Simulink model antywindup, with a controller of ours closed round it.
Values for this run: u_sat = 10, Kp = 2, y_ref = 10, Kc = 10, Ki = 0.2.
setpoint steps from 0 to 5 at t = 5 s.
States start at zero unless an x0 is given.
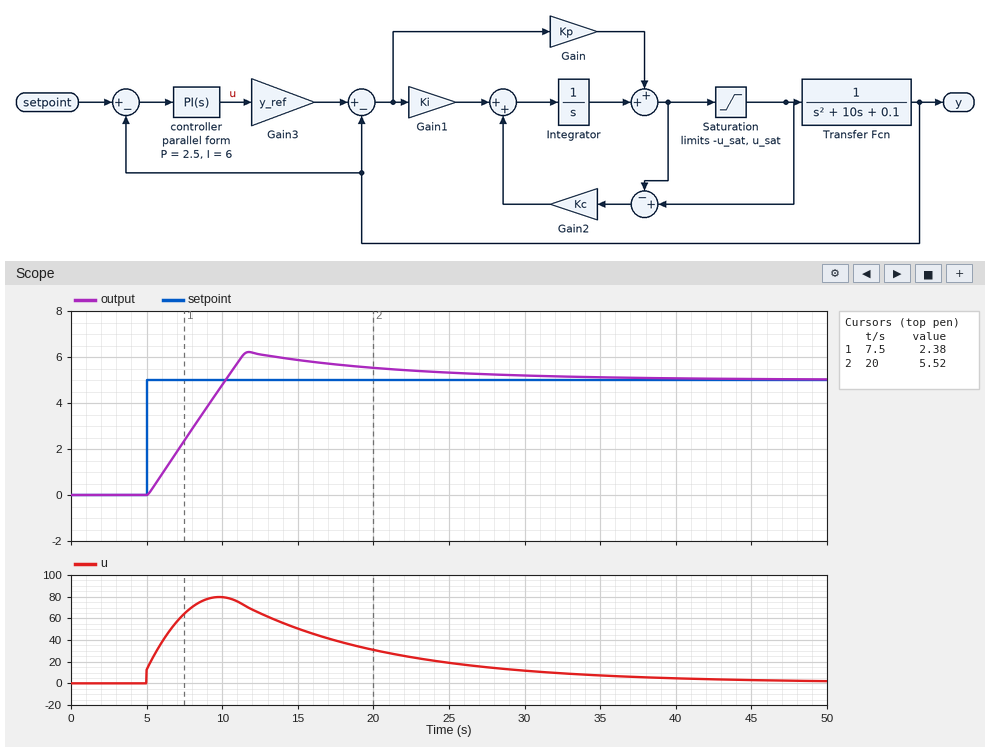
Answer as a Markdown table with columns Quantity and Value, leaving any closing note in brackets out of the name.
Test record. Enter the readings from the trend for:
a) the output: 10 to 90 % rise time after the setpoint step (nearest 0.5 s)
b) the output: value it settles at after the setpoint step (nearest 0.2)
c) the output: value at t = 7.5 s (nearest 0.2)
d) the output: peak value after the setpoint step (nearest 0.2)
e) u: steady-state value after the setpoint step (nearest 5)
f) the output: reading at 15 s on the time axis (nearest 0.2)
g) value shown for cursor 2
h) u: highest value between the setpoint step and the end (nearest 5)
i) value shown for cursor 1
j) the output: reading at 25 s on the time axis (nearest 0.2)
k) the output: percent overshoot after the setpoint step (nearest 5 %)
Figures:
| Quantity | Value |
|---|---|
| the output: 10 to 90 % rise time after the setpoint step | 4.0 s |
| the output: value it settles at after the setpoint step | 5.0 |
| the output: value at t = 7.5 s | 2.4 |
| the output: peak value after the setpoint step | 6.2 |
| u: steady-state value after the setpoint step | 0 |
| the output: reading at 15 s on the time axis | 5.8 |
| value shown for cursor 2 | 5.52 |
| u: highest value between the setpoint step and the end | 80 |
| value shown for cursor 1 | 2.38 |
| the output: reading at 25 s on the time axis | 5.4 |
| the output: percent overshoot after the setpoint step | 25 % |
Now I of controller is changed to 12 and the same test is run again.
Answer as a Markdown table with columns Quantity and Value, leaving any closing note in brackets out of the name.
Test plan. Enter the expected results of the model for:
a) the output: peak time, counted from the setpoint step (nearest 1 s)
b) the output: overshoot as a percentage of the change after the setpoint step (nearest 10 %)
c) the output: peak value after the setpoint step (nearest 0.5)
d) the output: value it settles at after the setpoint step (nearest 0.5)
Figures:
| Quantity | Value |
|---|---|
| the output: peak time, counted from the setpoint step | 7 s |
| the output: overshoot as a percentage of the change after the setpoint step | 30 % |
| the output: peak value after the setpoint step | 6.5 |
| the output: value it settles at after the setpoint step | 5.0 |
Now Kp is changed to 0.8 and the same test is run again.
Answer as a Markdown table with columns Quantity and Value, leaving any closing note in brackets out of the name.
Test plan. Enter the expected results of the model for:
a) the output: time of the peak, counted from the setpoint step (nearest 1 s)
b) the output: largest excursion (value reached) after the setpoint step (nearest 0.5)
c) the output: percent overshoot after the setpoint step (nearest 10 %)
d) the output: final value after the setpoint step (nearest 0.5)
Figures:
| Quantity | Value |
|---|---|
| the output: time of the peak, counted from the setpoint step | 8 s |
| the output: largest excursion (value reached) after the setpoint step | 7.5 |
| the output: percent overshoot after the setpoint step | 50 % |
| the output: final value after the setpoint step | 5.0 |
